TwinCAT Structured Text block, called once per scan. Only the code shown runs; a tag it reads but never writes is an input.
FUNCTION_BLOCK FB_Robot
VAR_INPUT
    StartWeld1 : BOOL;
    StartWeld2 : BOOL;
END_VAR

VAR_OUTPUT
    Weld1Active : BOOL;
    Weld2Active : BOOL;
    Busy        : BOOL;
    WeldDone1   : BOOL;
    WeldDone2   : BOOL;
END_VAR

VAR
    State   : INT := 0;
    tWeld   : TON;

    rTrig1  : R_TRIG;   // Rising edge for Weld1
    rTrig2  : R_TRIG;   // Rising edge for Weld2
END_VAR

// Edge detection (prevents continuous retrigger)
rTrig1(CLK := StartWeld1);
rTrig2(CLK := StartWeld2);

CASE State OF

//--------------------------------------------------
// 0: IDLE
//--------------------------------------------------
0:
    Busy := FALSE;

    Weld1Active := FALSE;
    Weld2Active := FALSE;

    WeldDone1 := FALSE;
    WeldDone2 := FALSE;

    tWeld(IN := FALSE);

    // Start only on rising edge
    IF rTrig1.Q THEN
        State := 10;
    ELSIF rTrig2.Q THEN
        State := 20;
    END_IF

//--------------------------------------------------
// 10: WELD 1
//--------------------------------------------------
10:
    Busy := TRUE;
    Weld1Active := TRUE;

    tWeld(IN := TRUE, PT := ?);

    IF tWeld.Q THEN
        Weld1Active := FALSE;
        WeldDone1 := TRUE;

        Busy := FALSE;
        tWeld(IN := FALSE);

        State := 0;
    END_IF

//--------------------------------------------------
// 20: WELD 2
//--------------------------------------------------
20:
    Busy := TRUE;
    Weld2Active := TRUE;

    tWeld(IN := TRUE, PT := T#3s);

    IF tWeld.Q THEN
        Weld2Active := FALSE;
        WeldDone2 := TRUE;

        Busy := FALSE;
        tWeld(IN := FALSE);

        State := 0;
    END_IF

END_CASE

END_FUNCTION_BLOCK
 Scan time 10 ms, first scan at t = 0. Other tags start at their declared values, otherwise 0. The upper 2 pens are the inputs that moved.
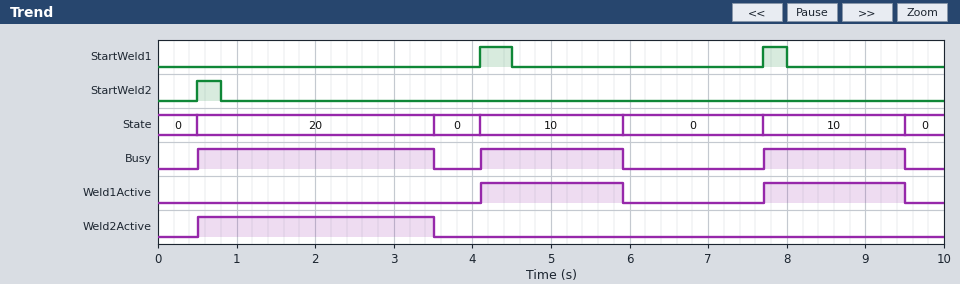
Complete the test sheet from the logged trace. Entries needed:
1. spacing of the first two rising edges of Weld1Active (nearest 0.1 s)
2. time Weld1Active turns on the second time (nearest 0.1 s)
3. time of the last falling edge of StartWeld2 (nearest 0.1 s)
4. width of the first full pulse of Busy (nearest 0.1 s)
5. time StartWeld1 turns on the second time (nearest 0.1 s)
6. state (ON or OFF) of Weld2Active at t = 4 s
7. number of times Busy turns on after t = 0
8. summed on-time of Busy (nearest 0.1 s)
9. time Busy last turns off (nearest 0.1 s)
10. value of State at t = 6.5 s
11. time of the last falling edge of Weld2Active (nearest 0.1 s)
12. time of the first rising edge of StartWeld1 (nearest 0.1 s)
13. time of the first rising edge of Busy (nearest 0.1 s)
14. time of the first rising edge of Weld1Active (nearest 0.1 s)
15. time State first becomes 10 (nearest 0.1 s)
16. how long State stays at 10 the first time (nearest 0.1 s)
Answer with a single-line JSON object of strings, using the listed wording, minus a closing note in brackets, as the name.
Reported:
{"spacing of the first two rising edges of Weld1Active": "3.6 s", "time Weld1Active turns on the second time": "7.7 s", "time of the last falling edge of StartWeld2": "0.8 s", "width of the first full pulse of Busy": "3.0 s", "time StartWeld1 turns on the second time": "7.7 s", "state (ON or OFF) of Weld2Active at t = 4 s": "OFF", "number of times Busy turns on after t = 0": "3", "summed on-time of Busy": "6.6 s", "time Busy last turns off": "9.5 s", "value of State at t = 6.5 s": "0", "time of the last falling edge of Weld2Active": "3.5 s", "time of the first rising edge of StartWeld1": "4.1 s", "time of the first rising edge of Busy": "0.5 s", "time of the first rising edge of Weld1Active": "4.1 s", "time State first becomes 10": "4.1 s", "how long State stays at 10 the first time": "1.8 s"}
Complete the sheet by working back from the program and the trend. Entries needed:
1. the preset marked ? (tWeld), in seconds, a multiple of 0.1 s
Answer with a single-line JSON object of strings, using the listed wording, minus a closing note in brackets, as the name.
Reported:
{"the preset marked ? (tWeld), in seconds, a multiple of 0.1 s": "1.8 s"}
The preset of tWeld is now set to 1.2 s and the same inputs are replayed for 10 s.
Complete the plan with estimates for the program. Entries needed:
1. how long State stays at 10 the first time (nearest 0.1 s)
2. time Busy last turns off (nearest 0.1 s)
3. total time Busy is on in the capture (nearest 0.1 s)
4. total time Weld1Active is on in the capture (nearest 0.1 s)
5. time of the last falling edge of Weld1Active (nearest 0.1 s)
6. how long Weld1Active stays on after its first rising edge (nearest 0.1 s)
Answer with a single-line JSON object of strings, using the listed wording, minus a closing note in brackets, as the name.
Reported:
{"how long State stays at 10 the first time": "1.2 s", "time Busy last turns off": "8.9 s", "total time Busy is on in the capture": "5.4 s", "total time Weld1Active is on in the capture": "2.4 s", "time of the last falling edge of Weld1Active": "8.9 s", "how long Weld1Active stays on after its first rising edge": "1.2 s"}
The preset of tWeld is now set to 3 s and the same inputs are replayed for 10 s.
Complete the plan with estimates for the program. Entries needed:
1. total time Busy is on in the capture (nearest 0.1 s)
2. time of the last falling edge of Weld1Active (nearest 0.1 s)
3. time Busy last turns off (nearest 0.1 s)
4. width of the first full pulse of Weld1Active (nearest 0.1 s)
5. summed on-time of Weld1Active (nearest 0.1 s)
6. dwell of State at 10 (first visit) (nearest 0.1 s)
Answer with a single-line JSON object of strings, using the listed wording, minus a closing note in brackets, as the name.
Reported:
{"total time Busy is on in the capture": "8.3 s", "time of the last falling edge of Weld1Active": "7.1 s", "time Busy last turns off": "7.1 s", "width of the first full pulse of Weld1Active": "3.0 s", "summed on-time of Weld1Active": "5.3 s", "dwell of State at 10 (first visit)": "3.0 s"}
